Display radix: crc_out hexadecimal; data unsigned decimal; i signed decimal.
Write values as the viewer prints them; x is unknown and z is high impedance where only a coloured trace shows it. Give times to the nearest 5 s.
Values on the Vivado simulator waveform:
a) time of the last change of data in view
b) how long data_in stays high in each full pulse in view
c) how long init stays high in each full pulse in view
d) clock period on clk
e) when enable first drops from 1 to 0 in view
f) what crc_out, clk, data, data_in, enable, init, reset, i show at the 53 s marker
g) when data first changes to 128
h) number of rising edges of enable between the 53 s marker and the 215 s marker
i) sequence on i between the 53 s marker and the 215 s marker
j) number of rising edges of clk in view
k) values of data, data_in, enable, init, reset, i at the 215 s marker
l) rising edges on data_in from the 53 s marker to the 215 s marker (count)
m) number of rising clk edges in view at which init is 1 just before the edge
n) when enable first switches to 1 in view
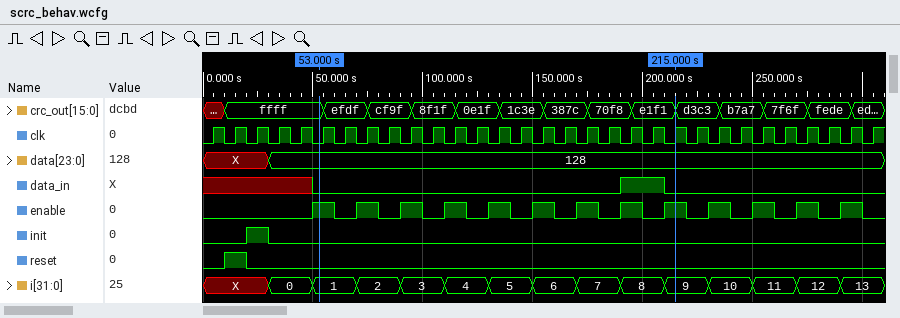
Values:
30 s
20 s
10 s
10 s
60 s
crc_out=ffff, clk=0, data=128, data_in=0, enable=1, init=0, reset=0, i=1
30 s
8
1, 2, 3, 4, 5, 6, 7, 8, 9
31
data=128, data_in=0, enable=1, init=0, reset=0, i=9
1
1
50 s
